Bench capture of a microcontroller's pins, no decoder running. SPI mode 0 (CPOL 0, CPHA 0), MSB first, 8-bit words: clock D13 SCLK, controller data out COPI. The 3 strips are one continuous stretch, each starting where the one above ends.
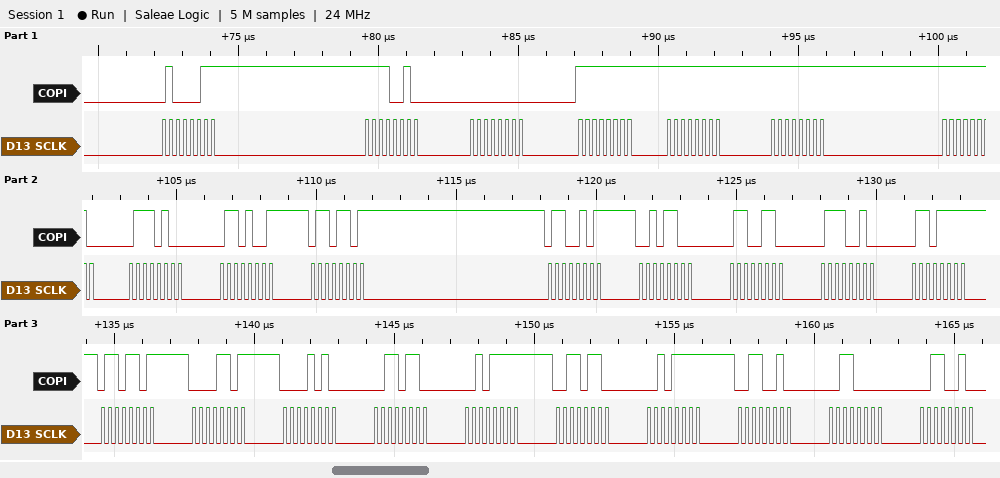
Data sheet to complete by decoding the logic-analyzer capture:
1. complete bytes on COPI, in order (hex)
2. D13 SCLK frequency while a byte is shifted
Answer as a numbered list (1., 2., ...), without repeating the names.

1. 43 F2 00 FF FF FF FE 74 69 6D 65 2C 66 72 6F 6D 0D 0A 36 2F 36 2F 32 30 32
2. 4 MHz
